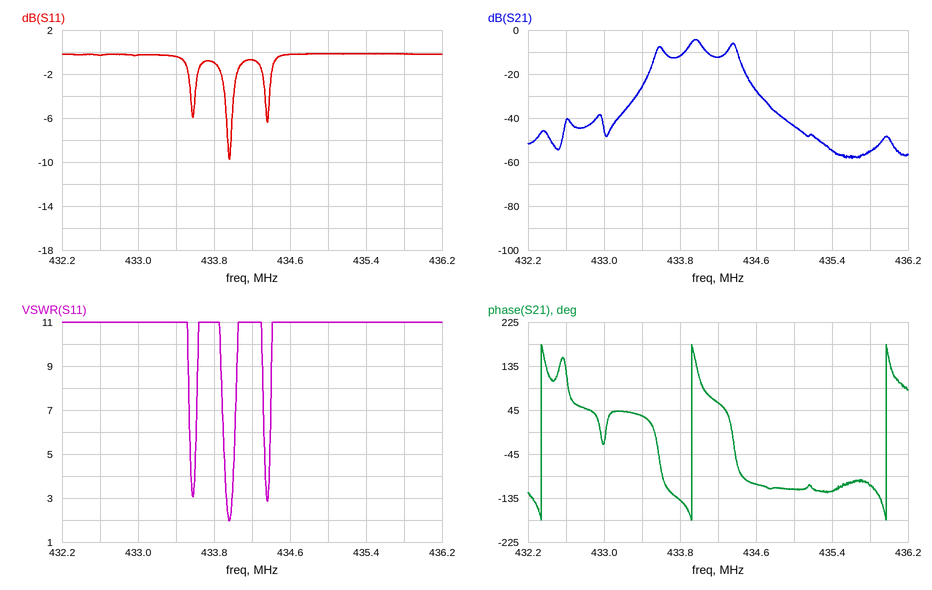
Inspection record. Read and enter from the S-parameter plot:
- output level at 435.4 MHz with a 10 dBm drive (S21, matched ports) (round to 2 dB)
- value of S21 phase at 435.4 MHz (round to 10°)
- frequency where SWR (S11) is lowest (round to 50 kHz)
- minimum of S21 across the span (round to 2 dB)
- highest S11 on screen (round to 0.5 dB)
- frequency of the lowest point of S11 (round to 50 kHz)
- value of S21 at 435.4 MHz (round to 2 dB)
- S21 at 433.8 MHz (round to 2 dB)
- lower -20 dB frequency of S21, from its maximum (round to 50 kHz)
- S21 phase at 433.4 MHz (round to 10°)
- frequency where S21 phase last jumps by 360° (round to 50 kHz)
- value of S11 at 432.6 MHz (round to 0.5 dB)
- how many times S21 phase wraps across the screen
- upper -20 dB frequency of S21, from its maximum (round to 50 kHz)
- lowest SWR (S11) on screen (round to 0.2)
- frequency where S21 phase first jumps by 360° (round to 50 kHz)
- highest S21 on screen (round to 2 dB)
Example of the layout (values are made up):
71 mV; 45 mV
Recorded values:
-44 dBm; -120°; 433.95 MHz; -58 dB; 0.0 dB; 433.95 MHz; -54 dB; -12 dB; 433.40 MHz; 30°; 435.95 MHz; -0.5 dB; 3; 434.55 MHz; 2.0; 432.35 MHz; -4 dB
